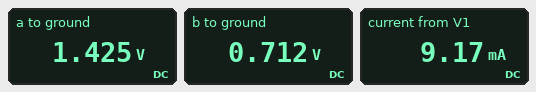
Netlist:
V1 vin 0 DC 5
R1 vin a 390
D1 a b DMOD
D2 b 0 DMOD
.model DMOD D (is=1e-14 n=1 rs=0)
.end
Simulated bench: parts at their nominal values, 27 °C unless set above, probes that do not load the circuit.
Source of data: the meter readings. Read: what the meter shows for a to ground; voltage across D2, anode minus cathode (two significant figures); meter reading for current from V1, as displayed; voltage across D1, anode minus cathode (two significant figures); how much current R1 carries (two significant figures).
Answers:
1.425 V
710 mV
9.17 mA
710 mV
9.2 mA
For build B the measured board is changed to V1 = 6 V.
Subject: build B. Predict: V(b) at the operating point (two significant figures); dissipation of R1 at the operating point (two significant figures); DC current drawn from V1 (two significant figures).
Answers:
720 mV
53 mW
12 mA
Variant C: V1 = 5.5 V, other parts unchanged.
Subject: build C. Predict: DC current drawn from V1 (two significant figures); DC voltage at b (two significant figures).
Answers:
10 mA
720 mV
